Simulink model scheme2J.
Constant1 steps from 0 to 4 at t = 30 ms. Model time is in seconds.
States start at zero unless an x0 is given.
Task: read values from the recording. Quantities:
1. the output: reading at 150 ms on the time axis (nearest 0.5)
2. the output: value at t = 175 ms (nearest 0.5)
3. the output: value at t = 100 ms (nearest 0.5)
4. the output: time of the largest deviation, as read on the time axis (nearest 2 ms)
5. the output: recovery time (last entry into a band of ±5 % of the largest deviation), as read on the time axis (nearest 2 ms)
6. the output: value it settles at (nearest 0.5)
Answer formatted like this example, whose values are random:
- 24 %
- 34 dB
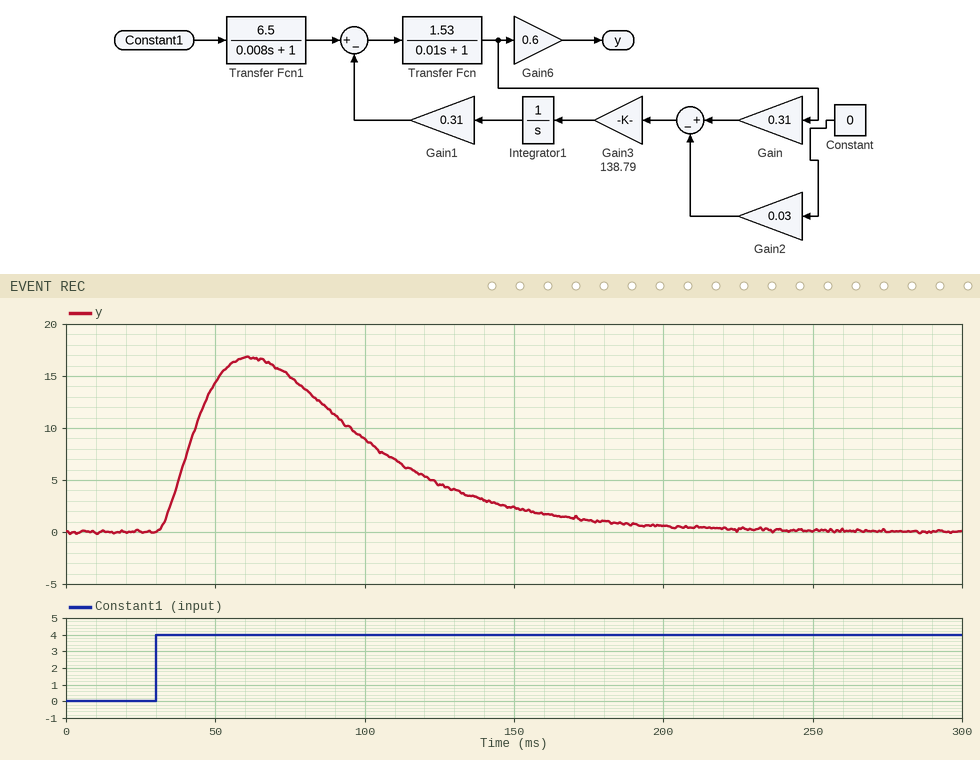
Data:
- 2.5
- 1.0
- 9.0
- 62 ms
- 186 ms
- 0.0
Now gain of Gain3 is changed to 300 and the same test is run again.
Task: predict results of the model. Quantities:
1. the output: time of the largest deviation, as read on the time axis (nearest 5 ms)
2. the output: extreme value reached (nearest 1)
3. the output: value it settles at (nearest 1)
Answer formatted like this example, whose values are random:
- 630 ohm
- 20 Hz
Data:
- 55 ms
- 14
- 0
